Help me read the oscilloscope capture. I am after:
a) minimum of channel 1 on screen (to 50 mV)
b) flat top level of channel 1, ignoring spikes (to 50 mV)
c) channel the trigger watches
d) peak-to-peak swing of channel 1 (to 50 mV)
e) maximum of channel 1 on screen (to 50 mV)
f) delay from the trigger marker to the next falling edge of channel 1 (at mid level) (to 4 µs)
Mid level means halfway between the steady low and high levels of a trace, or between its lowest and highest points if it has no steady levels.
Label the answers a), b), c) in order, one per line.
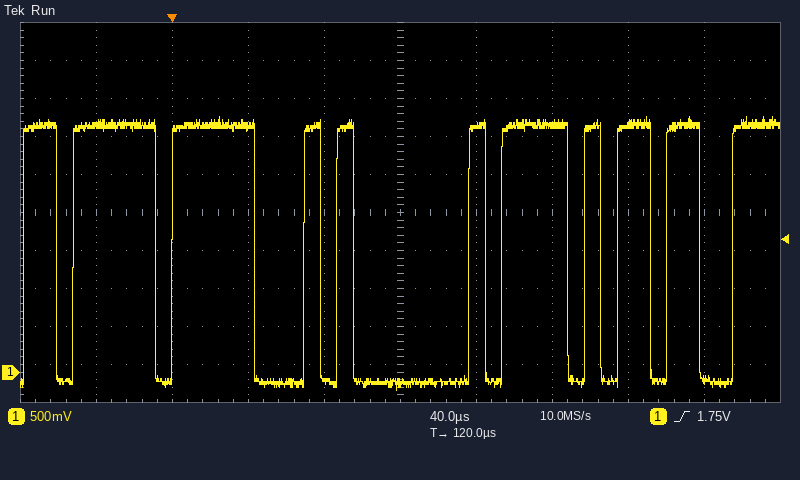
a) -250 mV
b) 3.25 V
c) channel 1
d) 3.60 V
e) 3.35 V
f) 44 µs
